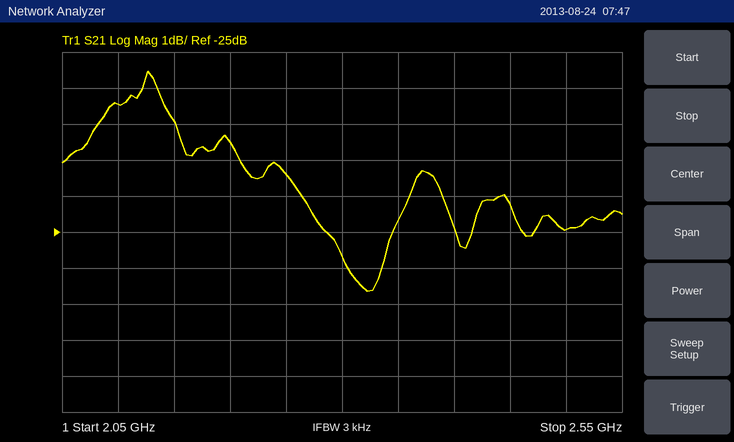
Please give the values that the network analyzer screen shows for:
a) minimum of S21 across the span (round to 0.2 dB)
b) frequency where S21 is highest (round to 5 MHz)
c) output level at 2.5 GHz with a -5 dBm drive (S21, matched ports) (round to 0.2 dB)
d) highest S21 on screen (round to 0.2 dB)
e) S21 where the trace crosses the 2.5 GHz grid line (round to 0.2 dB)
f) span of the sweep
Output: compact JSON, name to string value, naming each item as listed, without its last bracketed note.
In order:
{"minimum of S21 across the span": "-26.6 dB", "frequency where S21 is highest": "2.125 GHz", "output level at 2.5 GHz with a -5 dBm drive (S21, matched ports)": "-30.0 dBm", "highest S21 on screen": "-20.6 dB", "S21 where the trace crosses the 2.5 GHz grid line": "-25.0 dB", "span of the sweep": "500 MHz"}
